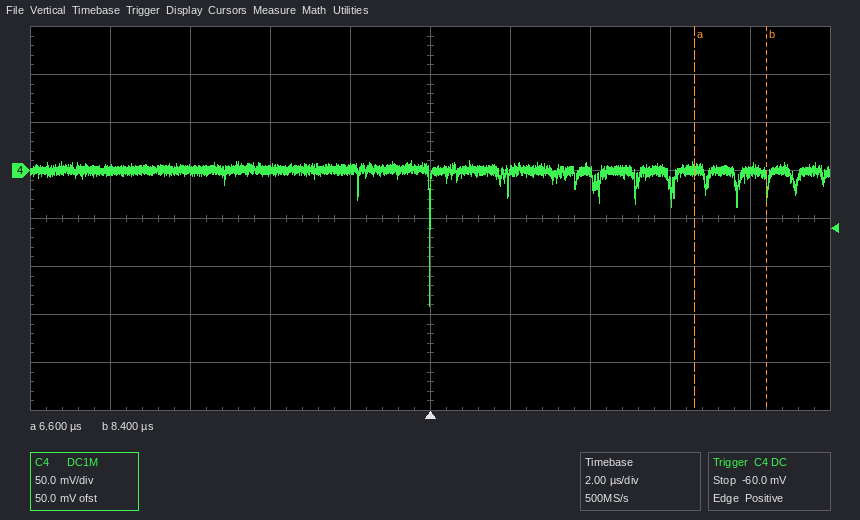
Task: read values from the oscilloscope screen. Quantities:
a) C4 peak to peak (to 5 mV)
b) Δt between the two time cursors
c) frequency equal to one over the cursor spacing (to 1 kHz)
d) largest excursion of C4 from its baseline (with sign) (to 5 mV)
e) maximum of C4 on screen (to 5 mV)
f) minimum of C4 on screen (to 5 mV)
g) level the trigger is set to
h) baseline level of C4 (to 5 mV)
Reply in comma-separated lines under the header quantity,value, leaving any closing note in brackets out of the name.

quantity,value
C4 peak to peak,150 mV
Δt between the two time cursors,1.8 µs
frequency equal to one over the cursor spacing,556 kHz
largest excursion of C4 from its baseline (with sign),-140 mV
maximum of C4 on screen,10 mV
minimum of C4 on screen,-140 mV
level the trigger is set to,-60.0 mV
baseline level of C4,0 mV
